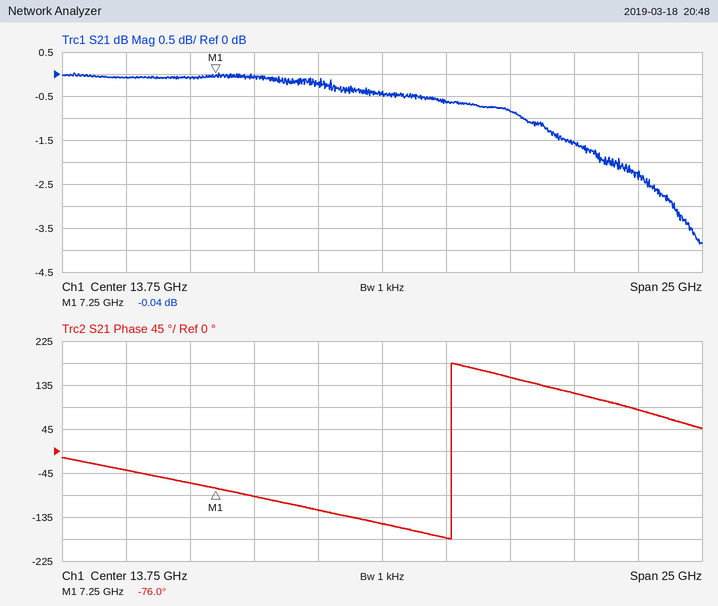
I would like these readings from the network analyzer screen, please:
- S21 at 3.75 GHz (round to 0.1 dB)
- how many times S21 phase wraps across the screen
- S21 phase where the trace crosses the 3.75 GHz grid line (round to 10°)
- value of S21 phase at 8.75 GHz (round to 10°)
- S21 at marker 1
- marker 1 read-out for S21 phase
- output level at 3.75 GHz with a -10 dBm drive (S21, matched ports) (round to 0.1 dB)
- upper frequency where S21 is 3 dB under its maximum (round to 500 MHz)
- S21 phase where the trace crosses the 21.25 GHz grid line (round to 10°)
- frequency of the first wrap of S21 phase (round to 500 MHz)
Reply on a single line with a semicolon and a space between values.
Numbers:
-0.1 dB; 1; -40°; -90°; -0.04 dB; -76.0°; -10.1 dBm; 25.0 GHz; 120°; 16.5 GHz
